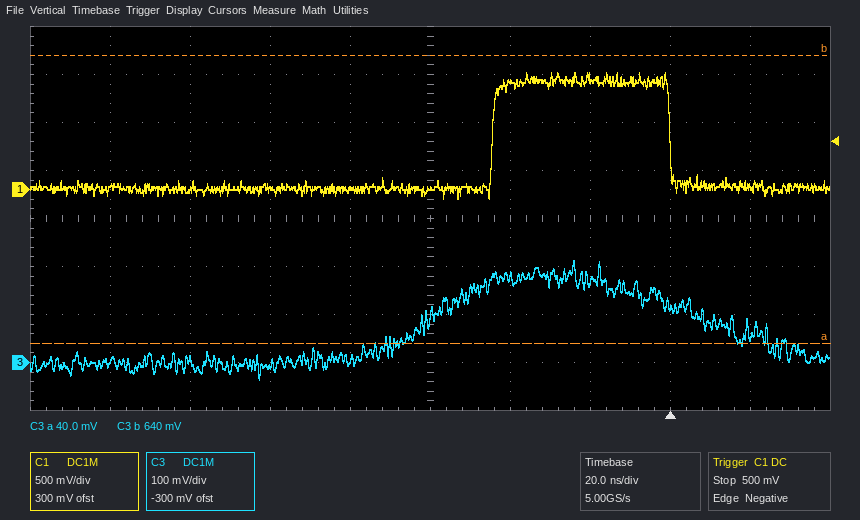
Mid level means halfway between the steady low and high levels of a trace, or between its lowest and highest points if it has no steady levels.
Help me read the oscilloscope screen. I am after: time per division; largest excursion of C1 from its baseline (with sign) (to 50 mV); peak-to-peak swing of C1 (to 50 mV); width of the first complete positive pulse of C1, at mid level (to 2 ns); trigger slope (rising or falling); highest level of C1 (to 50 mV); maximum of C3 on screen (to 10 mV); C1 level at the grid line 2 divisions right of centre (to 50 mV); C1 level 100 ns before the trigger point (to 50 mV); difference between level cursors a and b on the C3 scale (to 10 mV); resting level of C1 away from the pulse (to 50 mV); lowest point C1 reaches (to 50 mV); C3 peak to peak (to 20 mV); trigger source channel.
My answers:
20 ns
+1.20 V
1.30 V
44 ns
falling
1.20 V
210 mV
1.15 V
0 mV
600 mV
0 mV
-100 mV
240 mV
C1
